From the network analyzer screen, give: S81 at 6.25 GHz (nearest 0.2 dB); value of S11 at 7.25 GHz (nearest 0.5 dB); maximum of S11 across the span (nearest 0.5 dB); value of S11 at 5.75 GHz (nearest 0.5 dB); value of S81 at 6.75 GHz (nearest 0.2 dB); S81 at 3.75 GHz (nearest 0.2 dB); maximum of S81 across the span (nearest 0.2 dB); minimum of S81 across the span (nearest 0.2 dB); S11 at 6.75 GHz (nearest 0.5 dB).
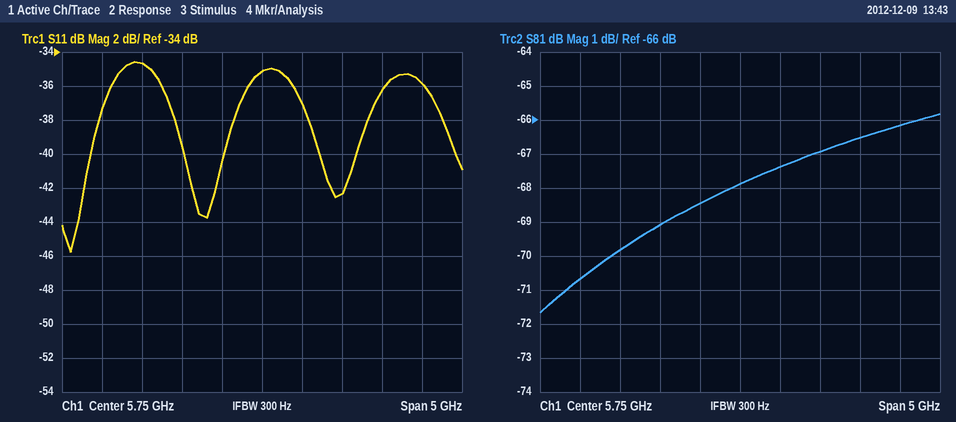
-67.4 dB
-36.5 dB
-34.5 dB
-35.0 dB
-67.0 dB
-70.6 dB
-65.8 dB
-71.6 dB
-42.5 dB
